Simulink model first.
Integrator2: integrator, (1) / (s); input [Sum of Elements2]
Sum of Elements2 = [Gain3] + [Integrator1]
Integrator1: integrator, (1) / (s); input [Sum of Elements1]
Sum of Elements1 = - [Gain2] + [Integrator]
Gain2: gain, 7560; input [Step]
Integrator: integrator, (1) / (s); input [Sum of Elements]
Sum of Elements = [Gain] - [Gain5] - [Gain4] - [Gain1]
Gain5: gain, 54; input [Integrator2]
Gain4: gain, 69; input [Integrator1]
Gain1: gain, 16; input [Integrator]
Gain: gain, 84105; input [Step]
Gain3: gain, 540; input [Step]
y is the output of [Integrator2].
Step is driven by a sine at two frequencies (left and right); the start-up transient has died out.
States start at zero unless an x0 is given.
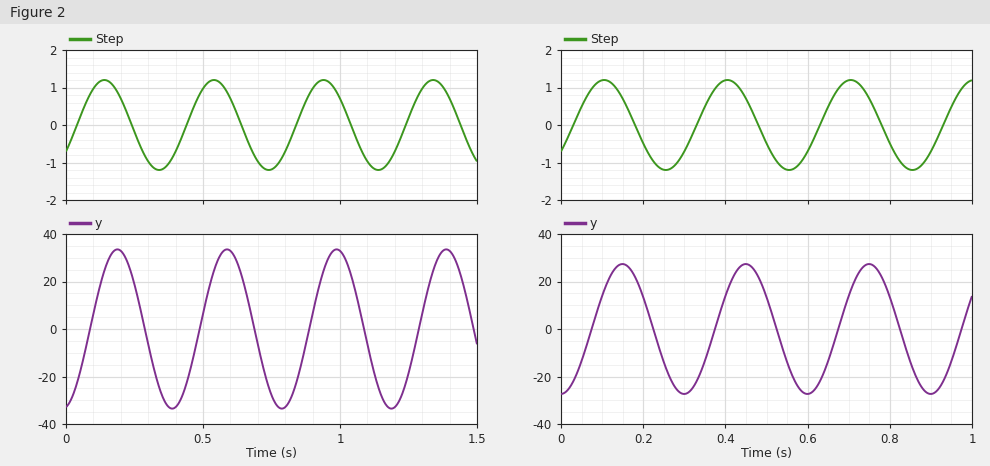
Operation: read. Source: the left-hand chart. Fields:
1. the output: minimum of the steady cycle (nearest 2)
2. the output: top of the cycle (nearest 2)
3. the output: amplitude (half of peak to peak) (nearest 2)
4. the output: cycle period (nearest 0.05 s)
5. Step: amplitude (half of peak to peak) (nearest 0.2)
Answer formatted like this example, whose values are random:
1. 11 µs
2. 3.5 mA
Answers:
1. -34
2. 34
3. 34
4. 0.40 s
5. 1.2
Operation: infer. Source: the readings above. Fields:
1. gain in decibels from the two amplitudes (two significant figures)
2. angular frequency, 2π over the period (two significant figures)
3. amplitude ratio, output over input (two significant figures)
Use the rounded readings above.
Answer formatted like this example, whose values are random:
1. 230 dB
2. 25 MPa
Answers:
1. 29 dB
2. 16 rad/s
3. 28
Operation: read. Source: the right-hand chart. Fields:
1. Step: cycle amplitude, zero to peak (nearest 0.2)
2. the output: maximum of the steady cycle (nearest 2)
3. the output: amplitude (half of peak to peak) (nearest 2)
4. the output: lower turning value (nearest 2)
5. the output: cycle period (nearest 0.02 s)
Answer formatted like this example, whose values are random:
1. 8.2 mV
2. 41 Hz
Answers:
1. 1.2
2. 28
3. 28
4. -28
5. 0.30 s
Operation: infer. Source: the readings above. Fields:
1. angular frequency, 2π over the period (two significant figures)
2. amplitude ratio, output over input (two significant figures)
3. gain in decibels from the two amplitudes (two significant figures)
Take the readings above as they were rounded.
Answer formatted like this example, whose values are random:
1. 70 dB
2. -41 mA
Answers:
1. 21 rad/s
2. 23
3. 27 dB
